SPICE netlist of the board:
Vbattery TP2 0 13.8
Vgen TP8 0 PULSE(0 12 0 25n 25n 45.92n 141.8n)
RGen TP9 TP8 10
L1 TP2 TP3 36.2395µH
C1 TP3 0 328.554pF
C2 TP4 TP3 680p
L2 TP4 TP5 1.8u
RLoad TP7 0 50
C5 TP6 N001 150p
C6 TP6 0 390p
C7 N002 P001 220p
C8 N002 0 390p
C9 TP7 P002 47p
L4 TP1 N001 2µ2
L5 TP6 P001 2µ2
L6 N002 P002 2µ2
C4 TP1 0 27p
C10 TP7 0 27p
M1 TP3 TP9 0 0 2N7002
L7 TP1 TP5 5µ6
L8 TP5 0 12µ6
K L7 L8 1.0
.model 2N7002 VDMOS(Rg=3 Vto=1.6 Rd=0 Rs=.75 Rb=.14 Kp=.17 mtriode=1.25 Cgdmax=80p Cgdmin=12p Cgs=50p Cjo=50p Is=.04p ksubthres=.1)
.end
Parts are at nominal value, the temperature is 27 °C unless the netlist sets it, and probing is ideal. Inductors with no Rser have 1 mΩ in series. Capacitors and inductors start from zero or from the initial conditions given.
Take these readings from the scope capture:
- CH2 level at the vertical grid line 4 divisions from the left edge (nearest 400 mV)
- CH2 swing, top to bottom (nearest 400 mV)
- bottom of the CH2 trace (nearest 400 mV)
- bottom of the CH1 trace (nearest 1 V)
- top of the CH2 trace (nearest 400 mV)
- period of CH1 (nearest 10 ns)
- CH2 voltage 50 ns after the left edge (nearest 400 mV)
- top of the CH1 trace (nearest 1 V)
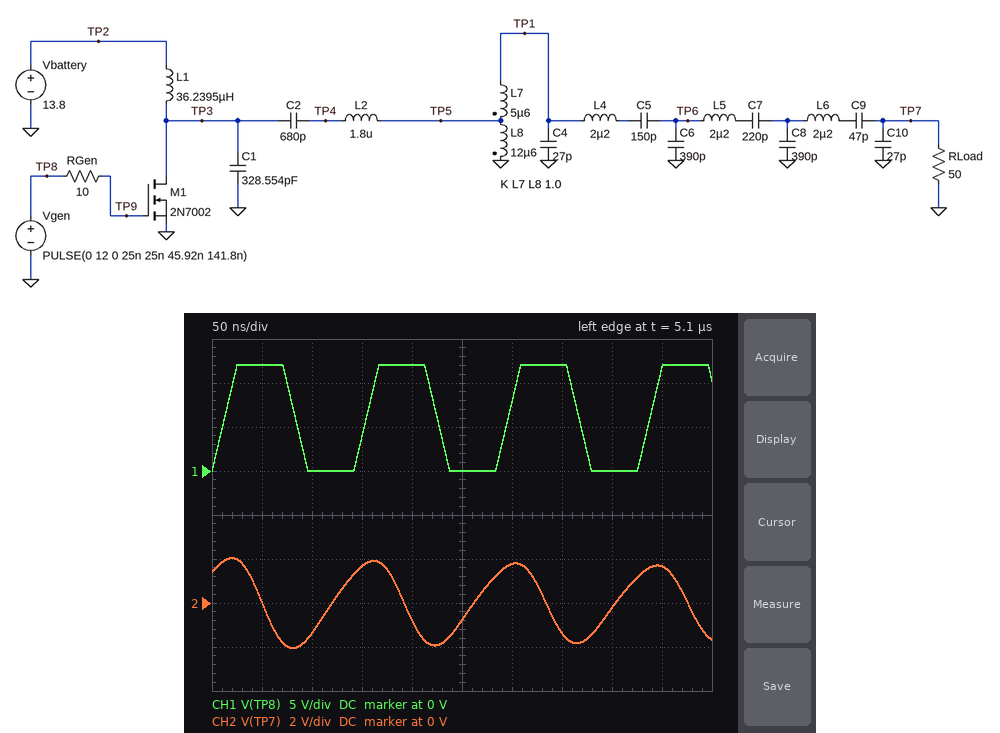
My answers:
-800 mV
4.0 V
-2.0 V
0 V
2.0 V
140 ns
0 V
12 V
